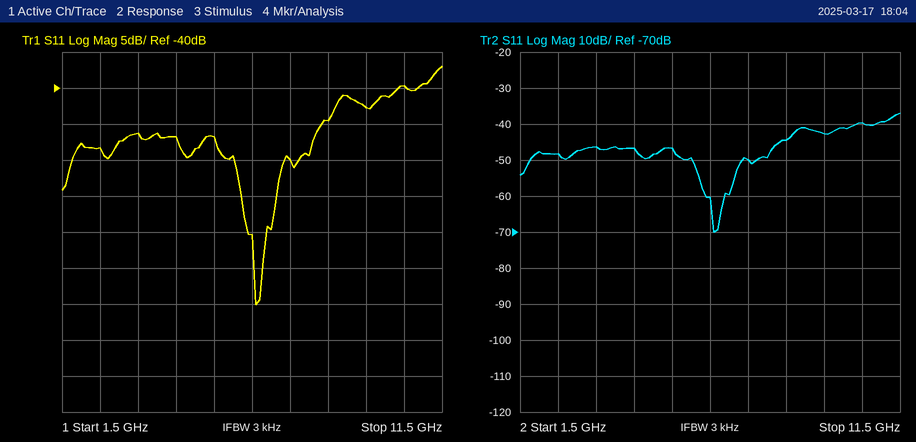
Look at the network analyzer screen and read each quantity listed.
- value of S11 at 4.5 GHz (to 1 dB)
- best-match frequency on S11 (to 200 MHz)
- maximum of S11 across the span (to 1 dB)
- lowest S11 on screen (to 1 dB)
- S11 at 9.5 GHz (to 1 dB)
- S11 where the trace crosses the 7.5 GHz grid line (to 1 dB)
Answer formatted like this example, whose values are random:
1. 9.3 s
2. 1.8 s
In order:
1. -47 dB
2. 6.6 GHz
3. -37 dB
4. -70 dB
5. -43 dB
6. -50 dB
